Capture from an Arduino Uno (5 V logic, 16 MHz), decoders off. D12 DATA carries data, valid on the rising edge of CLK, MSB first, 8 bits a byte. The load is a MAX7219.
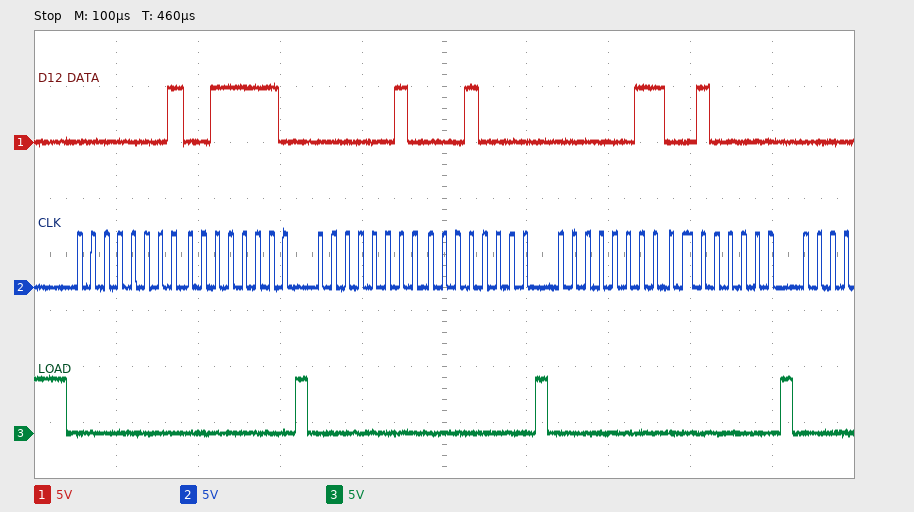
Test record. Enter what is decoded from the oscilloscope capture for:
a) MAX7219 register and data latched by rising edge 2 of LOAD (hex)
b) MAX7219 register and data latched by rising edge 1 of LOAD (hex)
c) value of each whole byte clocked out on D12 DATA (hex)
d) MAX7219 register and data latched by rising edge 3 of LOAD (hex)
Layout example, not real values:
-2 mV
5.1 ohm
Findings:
register 0x2, data 0x10
register 0x1, data 0x3E
01 3E 02 10 03 20
register 0x3, data 0x20
